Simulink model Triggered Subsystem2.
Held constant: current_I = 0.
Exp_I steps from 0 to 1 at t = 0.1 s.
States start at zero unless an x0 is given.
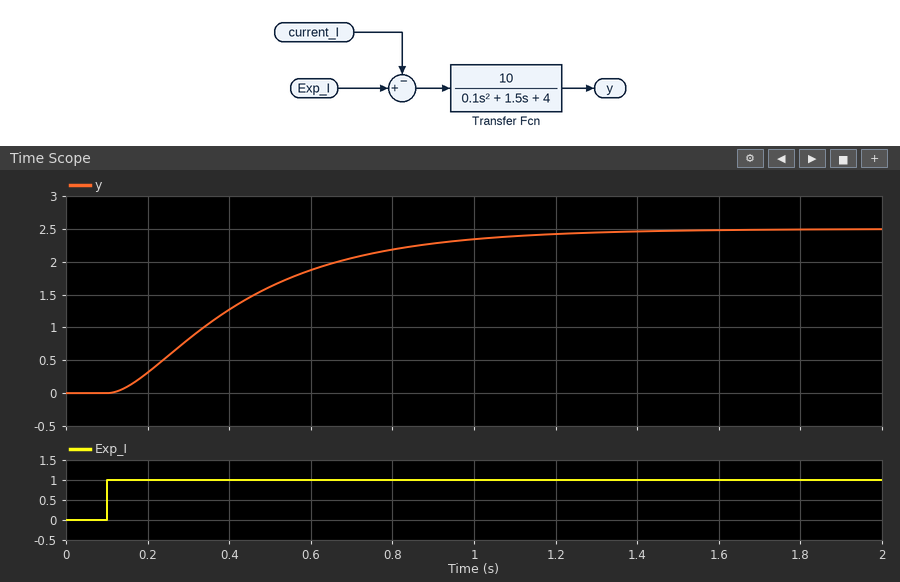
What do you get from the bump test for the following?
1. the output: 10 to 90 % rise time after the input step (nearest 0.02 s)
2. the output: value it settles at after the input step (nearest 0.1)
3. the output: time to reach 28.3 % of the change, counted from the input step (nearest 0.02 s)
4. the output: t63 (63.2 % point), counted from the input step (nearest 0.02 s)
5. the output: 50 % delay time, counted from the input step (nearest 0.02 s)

0.68 s
2.5
0.18 s
0.38 s
0.30 s
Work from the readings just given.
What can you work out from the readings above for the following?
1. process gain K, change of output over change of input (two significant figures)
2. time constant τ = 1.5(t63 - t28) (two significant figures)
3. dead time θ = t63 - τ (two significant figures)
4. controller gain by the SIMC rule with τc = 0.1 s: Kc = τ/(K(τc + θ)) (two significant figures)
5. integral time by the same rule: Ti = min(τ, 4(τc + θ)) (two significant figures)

2.5
0.30 s
0.080 s
0.67
0.30 s
